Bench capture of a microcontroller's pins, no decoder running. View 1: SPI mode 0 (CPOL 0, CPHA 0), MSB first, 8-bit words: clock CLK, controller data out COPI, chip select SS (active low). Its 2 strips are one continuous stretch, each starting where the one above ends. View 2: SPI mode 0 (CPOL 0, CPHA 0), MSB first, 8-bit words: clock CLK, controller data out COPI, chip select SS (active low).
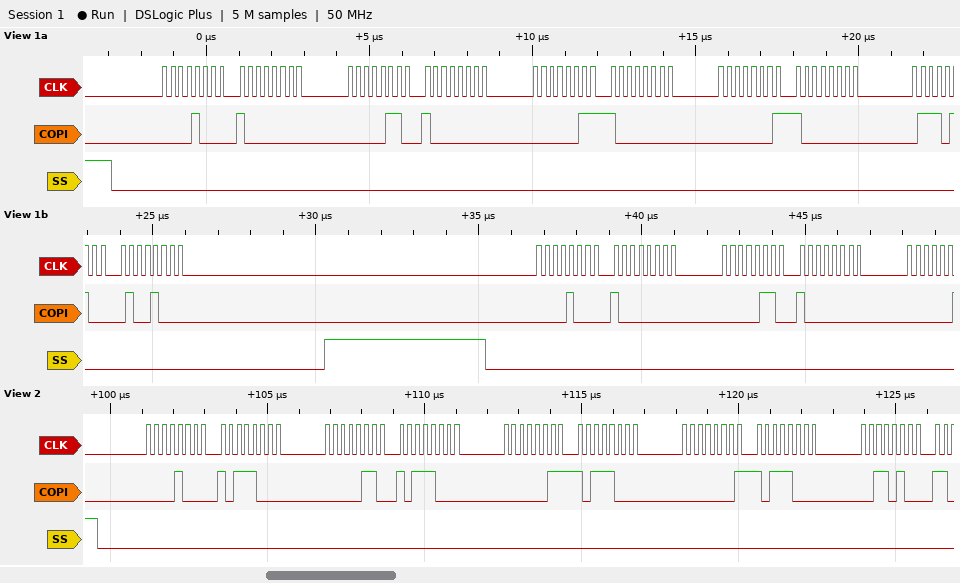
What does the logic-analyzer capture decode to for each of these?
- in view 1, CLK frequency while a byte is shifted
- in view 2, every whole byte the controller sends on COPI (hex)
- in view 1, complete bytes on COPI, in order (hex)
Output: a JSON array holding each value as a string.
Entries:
["4 MHz", "0x08 0xB8 0x06 0xB8 0x03 0xB8 0x01 0xB8 0x34", "08 80 06 80 03 80 01 80 74 48 08 80 06 80"]
